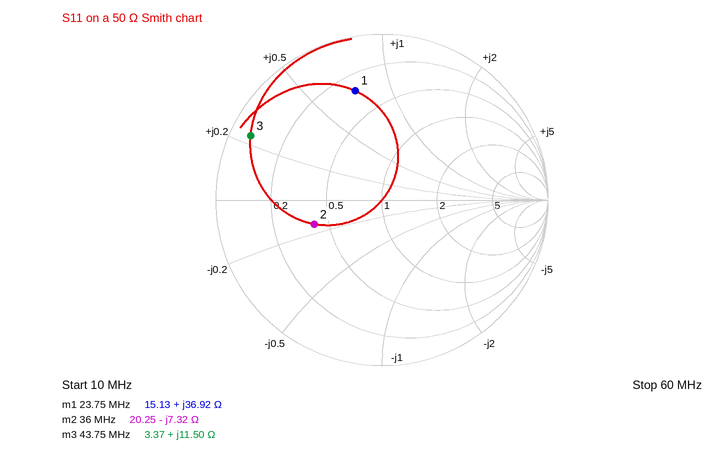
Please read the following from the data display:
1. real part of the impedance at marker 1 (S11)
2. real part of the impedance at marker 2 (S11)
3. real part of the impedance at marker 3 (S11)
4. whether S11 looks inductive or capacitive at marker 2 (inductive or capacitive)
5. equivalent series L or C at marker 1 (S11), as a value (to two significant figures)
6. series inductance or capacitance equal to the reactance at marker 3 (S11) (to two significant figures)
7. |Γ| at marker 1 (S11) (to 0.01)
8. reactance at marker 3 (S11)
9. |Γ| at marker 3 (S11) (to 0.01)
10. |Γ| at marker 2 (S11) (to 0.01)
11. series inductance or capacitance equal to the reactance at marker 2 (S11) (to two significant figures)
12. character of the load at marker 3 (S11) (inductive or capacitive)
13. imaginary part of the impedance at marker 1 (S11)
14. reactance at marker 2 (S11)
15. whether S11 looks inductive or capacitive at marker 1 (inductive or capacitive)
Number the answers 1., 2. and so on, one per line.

1. 15.13 Ω
2. 20.25 Ω
3. 3.37 Ω
4. capacitive
5. 250 nH
6. 42 nH
7. 0.68
8. +11.50 Ω
9. 0.88
10. 0.43
11. 600 pF
12. inductive
13. +36.92 Ω
14. -7.32 Ω
15. inductive
